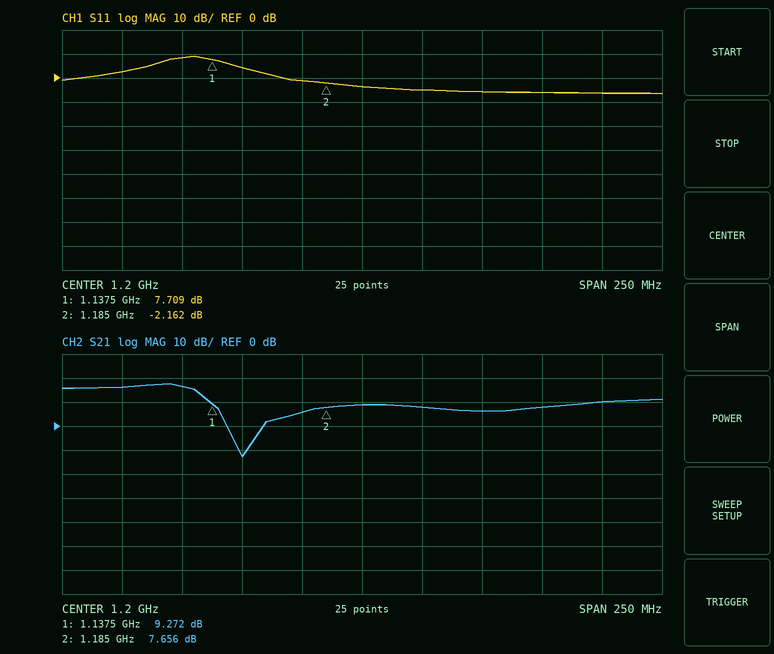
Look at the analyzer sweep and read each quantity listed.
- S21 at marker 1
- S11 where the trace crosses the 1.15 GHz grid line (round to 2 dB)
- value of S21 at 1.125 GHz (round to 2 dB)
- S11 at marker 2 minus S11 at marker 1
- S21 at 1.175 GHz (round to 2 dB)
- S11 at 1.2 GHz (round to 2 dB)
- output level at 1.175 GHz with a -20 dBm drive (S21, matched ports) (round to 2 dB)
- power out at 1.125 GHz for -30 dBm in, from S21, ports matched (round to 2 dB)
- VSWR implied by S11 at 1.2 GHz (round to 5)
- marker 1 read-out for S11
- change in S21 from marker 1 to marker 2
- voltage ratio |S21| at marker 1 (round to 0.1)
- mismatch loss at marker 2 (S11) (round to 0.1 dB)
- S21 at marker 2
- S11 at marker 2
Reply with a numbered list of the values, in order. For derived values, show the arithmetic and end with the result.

1. 9.272 dB
2. 4 dB
3. 16 dB
4. -2.162 − (7.709) = -9.871 dB
5. 6 dB
6. -4 dB
7. -20 dBm + (6 dB) = -14 dBm
8. -30 dBm + (16 dB) = -14 dBm
9. |Γ| = 10^(-4/20) = 0.6310; VSWR = (1 + 0.6310)/(1 − 0.6310) ≈ 4.42, so 5 to the nearest 5
10. 7.709 dB
11. 7.656 − (9.272) = -1.616 dB
12. 10^(9.272/20) ≈ 2.9
13. −10 log10(1 − 10^(-2.162/10)) ≈ 4.1 dB
14. 7.656 dB
15. -2.162 dB
